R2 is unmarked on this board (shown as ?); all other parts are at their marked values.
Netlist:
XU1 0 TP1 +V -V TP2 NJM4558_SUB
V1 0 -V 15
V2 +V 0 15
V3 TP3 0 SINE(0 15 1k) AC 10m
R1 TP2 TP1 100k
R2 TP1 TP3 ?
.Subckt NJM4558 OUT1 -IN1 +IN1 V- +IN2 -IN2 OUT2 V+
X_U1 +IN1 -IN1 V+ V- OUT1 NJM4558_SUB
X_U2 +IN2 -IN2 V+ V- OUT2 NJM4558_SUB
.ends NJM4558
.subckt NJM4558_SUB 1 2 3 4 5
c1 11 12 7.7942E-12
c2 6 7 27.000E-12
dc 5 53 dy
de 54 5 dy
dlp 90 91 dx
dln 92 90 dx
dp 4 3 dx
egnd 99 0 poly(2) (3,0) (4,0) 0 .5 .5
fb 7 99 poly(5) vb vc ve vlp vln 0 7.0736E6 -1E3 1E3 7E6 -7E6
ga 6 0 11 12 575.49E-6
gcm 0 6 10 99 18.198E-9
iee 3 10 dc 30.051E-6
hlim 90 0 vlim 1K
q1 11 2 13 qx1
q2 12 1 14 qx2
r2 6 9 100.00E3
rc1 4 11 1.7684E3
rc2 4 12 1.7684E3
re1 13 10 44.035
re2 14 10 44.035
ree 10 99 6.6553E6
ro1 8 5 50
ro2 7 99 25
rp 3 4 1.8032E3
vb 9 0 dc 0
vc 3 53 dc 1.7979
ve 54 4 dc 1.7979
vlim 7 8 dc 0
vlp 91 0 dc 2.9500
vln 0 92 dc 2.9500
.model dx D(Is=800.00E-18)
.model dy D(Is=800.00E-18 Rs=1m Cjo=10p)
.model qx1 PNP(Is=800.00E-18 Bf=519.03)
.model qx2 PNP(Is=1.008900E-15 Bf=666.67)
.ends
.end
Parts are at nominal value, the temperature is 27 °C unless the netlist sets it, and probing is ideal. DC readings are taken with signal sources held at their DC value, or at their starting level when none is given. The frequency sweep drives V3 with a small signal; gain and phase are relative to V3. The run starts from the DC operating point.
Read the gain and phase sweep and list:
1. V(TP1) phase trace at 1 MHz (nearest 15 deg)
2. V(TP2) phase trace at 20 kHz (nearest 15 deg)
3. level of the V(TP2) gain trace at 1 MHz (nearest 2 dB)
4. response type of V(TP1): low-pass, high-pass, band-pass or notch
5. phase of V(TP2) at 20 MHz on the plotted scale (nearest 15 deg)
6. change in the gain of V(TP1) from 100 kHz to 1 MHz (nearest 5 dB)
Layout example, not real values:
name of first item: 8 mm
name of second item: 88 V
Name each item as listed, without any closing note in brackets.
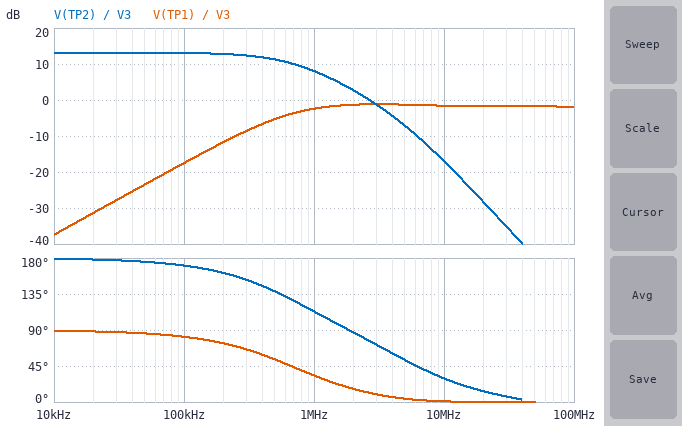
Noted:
V(TP1) phase trace at 1 MHz: 30 deg
V(TP2) phase trace at 20 kHz: 180 deg
level of the V(TP2) gain trace at 1 MHz: 8 dB
response type of V(TP1): low-pass, high-pass, band-pass or notch: high-pass
phase of V(TP2) at 20 MHz on the plotted scale: 15 deg
change in the gain of V(TP1) from 100 kHz to 1 MHz: 15 dB
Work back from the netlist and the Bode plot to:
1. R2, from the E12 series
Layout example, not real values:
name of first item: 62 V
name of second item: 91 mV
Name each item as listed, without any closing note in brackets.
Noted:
R2, from the E12 series: 22 kΩ
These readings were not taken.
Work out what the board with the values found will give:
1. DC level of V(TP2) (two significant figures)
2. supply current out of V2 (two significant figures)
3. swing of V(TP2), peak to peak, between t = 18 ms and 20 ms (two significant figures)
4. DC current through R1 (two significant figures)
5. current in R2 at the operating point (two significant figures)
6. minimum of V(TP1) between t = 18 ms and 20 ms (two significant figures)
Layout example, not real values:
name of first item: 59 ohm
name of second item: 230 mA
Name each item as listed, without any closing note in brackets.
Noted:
DC level of V(TP2): -36 mV
supply current out of V2: 17 mA
swing of V(TP2), peak to peak, between t = 18 ms and 20 ms: 28 V
DC current through R1: 300 nA
current in R2 at the operating point: 270 nA
minimum of V(TP1) between t = 18 ms and 20 ms: -9.8 V
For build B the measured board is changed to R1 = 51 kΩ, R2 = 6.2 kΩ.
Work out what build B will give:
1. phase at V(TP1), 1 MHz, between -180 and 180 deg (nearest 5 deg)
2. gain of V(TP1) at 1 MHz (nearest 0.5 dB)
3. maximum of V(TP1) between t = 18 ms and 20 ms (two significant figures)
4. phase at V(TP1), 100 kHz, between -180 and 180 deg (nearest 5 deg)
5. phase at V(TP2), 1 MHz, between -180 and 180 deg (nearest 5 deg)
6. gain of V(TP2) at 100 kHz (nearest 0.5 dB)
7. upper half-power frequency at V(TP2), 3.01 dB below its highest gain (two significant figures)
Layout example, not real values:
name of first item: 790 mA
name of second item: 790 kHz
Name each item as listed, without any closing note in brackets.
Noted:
phase at V(TP1), 1 MHz, between -180 and 180 deg: 20 deg
gain of V(TP1) at 1 MHz: -1.0 dB
maximum of V(TP1) between t = 18 ms and 20 ms: 12 V
phase at V(TP1), 100 kHz, between -180 and 180 deg: 75 deg
phase at V(TP2), 1 MHz, between -180 and 180 deg: 100 deg
gain of V(TP2) at 100 kHz: 18.0 dB
upper half-power frequency at V(TP2), 3.01 dB below its highest gain: 390 kHz
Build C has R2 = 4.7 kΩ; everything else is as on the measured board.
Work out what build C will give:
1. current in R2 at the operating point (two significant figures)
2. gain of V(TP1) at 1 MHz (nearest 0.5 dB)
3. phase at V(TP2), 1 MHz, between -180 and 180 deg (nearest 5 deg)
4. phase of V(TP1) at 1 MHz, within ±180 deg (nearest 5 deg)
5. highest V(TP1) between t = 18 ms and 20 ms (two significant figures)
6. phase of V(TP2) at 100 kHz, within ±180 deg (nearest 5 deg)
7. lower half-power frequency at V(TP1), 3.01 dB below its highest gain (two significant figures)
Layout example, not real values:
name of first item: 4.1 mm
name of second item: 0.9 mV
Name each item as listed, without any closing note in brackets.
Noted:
current in R2 at the operating point: 1.3 µA
gain of V(TP1) at 1 MHz: -0.5 dB
phase at V(TP2), 1 MHz, between -180 and 180 deg: 90 deg
phase of V(TP1) at 1 MHz, within ±180 deg: 10 deg
highest V(TP1) between t = 18 ms and 20 ms: 14 V
phase of V(TP2) at 100 kHz, within ±180 deg: 145 deg
lower half-power frequency at V(TP1), 3.01 dB below its highest gain: 150 kHz
